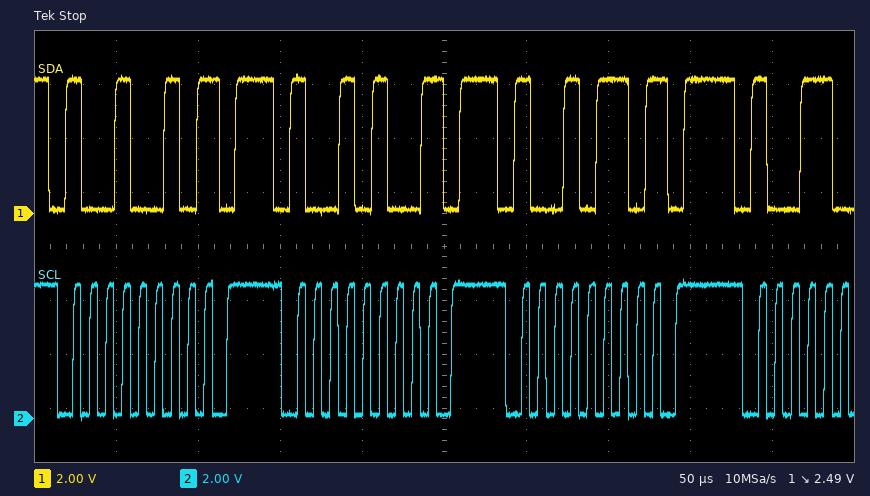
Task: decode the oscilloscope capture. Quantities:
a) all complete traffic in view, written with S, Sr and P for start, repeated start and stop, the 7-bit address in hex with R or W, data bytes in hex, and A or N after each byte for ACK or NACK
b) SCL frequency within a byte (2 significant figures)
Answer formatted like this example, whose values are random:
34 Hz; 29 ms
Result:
S 49W N P S 4AW N P S 4BW N P; 100 kHz
